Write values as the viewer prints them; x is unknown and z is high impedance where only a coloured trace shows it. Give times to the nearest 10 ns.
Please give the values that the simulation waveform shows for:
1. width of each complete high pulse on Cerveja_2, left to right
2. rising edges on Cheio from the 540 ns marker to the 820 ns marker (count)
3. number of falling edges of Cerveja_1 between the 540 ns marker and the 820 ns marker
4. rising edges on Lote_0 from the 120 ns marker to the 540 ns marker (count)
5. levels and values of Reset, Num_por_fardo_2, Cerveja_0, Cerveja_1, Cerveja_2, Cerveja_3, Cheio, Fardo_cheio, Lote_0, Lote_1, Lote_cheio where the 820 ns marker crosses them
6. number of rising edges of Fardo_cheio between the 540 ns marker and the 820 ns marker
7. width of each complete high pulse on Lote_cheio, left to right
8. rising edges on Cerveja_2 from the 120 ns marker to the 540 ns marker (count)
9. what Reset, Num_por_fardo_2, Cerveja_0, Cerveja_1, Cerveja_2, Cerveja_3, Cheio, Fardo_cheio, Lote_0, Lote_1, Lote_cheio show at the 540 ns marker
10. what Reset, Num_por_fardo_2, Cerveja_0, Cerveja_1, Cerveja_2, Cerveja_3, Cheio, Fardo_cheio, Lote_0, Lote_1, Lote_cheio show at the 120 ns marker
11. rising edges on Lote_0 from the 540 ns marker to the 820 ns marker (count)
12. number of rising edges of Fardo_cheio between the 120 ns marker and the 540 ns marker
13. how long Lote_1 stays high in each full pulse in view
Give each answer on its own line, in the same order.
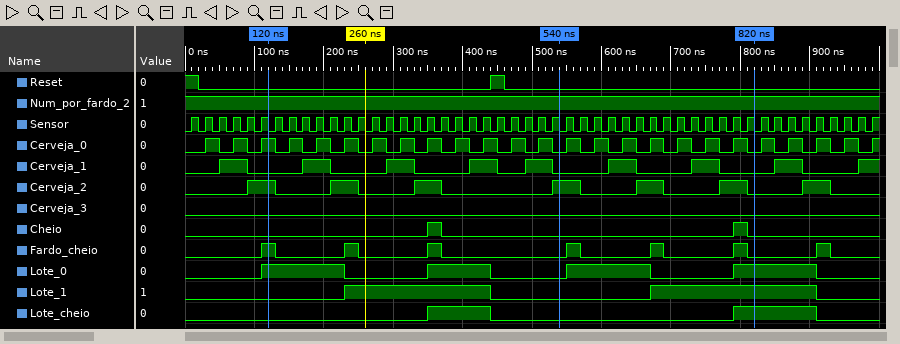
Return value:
40 ns, 40 ns, 40 ns, 40 ns, 40 ns, 40 ns, 40 ns
1
2
1
Reset=0, Num_por_fardo_2=1, Cerveja_0=0, Cerveja_1=0, Cerveja_2=0, Cerveja_3=0, Cheio=0, Fardo_cheio=0, Lote_0=1, Lote_1=1, Lote_cheio=1
3
90 ns, 120 ns
3
Reset=0, Num_por_fardo_2=1, Cerveja_0=0, Cerveja_1=0, Cerveja_2=1, Cerveja_3=0, Cheio=0, Fardo_cheio=0, Lote_0=0, Lote_1=0, Lote_cheio=0
Reset=0, Num_por_fardo_2=1, Cerveja_0=1, Cerveja_1=0, Cerveja_2=1, Cerveja_3=0, Cheio=0, Fardo_cheio=1, Lote_0=1, Lote_1=0, Lote_cheio=0
2
2
210 ns, 240 ns
